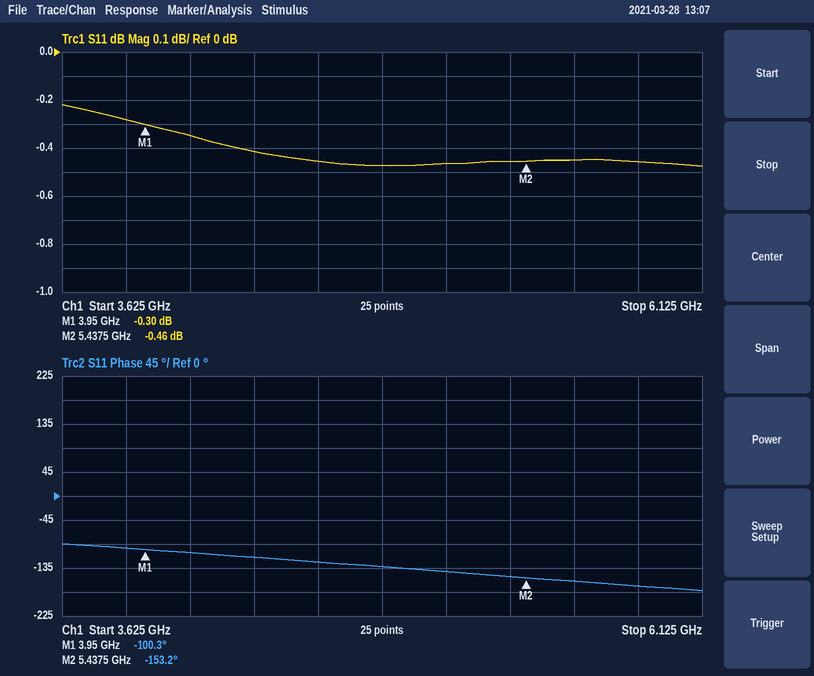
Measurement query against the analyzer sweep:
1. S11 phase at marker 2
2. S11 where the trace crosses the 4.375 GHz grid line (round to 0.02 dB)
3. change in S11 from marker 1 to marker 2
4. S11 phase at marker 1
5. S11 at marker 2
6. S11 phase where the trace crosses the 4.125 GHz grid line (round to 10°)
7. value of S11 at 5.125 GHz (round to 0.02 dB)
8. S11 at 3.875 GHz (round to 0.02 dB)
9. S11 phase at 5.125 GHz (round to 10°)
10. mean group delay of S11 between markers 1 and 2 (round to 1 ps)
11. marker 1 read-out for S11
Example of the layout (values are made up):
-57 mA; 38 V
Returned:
-153.2°; -0.42 dB; -0.16 dB; -100.3°; -0.46 dB; -110°; -0.46 dB; -0.28 dB; -140°; 99 ps; -0.30 dB
